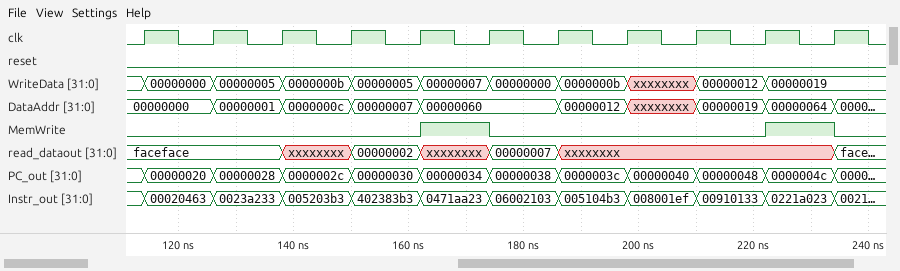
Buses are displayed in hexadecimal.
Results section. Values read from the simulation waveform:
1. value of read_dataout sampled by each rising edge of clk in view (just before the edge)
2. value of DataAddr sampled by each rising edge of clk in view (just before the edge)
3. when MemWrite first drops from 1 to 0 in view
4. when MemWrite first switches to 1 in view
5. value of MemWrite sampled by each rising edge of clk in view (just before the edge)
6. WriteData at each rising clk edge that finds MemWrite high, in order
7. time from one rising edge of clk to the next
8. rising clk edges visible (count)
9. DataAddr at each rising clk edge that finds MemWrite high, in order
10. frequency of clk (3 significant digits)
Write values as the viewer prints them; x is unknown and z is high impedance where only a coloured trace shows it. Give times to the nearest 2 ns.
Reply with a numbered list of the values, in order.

1. faceface, faceface, faceface, xxxxxxxx, 00000002, xxxxxxxx, 00000007, xxxxxxxx, xxxxxxxx, xxxxxxxx, xxxxxxxx
2. 00000000, 00000000, 00000001, 0000000c, 00000007, 00000060, 00000060, 00000012, xxxxxxxx, 00000019, 00000064
3. 174 ns
4. 162 ns
5. 0 0 0 0 0 1 0 0 0 0 1
6. 00000007, 00000019
7. 12 ns
8. 11
9. 00000060, 00000064
10. 83.3 MHz
